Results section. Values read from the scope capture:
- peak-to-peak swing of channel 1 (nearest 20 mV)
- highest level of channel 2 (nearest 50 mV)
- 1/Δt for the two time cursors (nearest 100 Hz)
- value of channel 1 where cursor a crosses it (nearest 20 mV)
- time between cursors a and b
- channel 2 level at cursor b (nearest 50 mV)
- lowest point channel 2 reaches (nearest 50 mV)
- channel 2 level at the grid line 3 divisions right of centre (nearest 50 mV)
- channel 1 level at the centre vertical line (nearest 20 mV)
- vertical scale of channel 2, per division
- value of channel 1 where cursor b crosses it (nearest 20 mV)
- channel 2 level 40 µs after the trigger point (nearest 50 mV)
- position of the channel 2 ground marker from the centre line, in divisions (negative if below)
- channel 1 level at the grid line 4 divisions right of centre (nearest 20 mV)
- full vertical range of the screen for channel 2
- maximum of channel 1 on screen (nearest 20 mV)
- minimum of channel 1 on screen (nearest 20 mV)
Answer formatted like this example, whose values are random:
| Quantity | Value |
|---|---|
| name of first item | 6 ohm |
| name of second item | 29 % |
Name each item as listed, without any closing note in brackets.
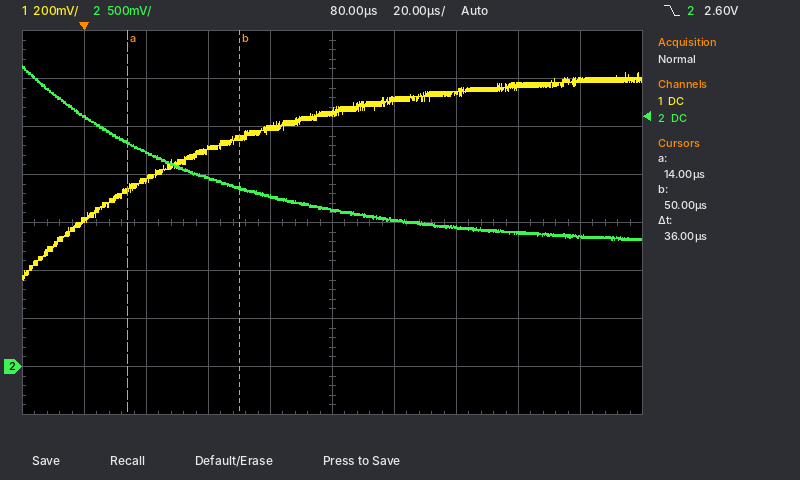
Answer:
| Quantity | Value |
|---|---|
| peak-to-peak swing of channel 1 | 860 mV |
| highest level of channel 2 | 3.15 V |
| 1/Δt for the two time cursors | 27.8 kHz |
| value of channel 1 where cursor a crosses it | 740 mV |
| time between cursors a and b | 36 µs |
| channel 2 level at cursor b | 1.85 V |
| lowest point channel 2 reaches | 1.30 V |
| channel 2 level at the grid line 3 divisions right of centre | 1.40 V |
| channel 1 level at the centre vertical line | 1.06 V |
| vertical scale of channel 2, per division | 500 mV |
| value of channel 1 where cursor b crosses it | 960 mV |
| channel 2 level 40 µs after the trigger point | 1.95 V |
| position of the channel 2 ground marker from the centre line, in divisions | -3.0 div |
| channel 1 level at the grid line 4 divisions right of centre | 1.20 V |
| full vertical range of the screen for channel 2 | 4 V |
| maximum of channel 1 on screen | 1.22 V |
| minimum of channel 1 on screen | 360 mV |
